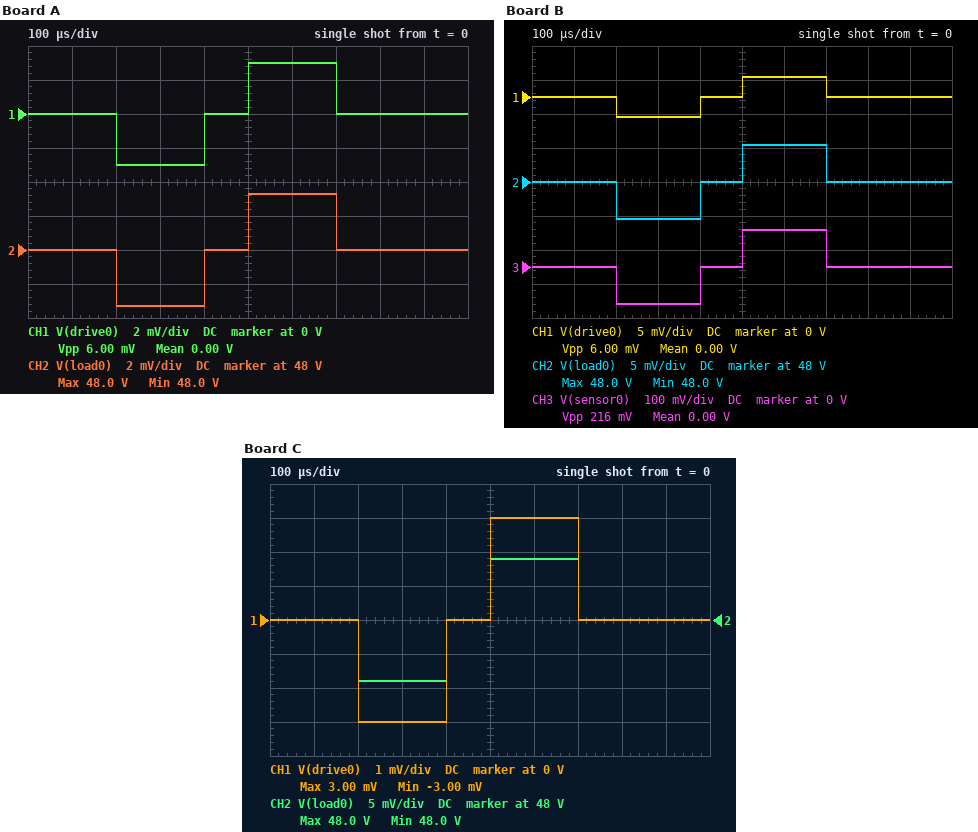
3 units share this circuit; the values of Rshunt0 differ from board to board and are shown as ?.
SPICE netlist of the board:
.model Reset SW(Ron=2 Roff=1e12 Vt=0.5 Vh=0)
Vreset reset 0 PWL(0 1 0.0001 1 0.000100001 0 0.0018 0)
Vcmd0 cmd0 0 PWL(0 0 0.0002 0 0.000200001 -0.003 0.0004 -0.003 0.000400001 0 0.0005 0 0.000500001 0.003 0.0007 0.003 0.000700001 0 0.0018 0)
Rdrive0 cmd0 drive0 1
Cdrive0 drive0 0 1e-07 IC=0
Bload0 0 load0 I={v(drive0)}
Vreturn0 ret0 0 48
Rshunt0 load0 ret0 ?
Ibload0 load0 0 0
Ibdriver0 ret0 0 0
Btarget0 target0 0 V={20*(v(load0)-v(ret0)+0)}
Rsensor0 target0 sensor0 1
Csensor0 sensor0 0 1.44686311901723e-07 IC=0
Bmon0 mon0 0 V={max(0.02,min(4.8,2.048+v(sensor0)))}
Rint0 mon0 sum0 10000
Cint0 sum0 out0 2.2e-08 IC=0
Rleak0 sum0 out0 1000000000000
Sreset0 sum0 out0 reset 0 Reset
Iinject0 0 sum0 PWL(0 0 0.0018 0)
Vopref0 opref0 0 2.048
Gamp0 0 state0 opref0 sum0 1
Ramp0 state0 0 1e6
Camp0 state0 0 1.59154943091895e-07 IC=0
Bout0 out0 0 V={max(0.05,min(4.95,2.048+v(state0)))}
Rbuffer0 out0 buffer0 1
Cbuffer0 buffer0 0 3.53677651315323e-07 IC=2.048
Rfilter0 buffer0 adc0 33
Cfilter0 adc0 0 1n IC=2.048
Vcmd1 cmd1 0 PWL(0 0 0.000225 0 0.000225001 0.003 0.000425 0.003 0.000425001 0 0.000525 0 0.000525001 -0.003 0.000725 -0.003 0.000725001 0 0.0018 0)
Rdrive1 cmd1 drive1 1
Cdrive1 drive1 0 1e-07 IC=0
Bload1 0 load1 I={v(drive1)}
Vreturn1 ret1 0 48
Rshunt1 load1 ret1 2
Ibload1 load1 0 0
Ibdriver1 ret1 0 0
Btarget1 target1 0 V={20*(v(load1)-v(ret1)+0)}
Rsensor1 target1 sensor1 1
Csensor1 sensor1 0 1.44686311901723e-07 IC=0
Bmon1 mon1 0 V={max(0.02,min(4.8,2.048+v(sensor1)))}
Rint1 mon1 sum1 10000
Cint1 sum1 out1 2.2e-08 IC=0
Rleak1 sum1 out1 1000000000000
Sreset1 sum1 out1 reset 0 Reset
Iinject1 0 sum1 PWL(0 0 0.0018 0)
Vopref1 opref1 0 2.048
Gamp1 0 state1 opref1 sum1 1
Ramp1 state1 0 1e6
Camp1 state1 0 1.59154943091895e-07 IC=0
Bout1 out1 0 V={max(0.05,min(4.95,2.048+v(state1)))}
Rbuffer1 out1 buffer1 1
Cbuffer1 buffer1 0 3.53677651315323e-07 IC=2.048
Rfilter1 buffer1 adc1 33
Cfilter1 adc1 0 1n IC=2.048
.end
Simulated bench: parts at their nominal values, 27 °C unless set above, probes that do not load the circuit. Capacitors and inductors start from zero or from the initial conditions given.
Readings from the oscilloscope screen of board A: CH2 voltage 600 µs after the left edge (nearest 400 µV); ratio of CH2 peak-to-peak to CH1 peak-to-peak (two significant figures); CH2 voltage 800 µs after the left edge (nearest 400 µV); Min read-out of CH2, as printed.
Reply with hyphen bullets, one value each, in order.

- 48.0032 V
- 1.1
- 48.0000 V
- 48.0 V
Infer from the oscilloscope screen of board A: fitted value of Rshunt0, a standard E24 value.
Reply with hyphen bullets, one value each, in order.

- 1.1 Ω
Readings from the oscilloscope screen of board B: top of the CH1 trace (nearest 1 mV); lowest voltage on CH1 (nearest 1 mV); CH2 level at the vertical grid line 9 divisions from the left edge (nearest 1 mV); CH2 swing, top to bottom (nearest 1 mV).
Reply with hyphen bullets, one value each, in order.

- 3 mV
- -3 mV
- 48.000 V
- 11 mV
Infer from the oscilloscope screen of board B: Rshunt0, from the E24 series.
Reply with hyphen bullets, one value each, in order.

- 1.8 Ω
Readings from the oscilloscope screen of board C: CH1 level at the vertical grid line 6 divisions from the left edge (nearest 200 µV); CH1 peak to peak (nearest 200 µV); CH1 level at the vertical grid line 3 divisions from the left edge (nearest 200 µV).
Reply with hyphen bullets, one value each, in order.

- 3.0 mV
- 6.0 mV
- -3.0 mV
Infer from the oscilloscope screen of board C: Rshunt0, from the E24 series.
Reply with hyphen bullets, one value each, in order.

- 3 Ω
